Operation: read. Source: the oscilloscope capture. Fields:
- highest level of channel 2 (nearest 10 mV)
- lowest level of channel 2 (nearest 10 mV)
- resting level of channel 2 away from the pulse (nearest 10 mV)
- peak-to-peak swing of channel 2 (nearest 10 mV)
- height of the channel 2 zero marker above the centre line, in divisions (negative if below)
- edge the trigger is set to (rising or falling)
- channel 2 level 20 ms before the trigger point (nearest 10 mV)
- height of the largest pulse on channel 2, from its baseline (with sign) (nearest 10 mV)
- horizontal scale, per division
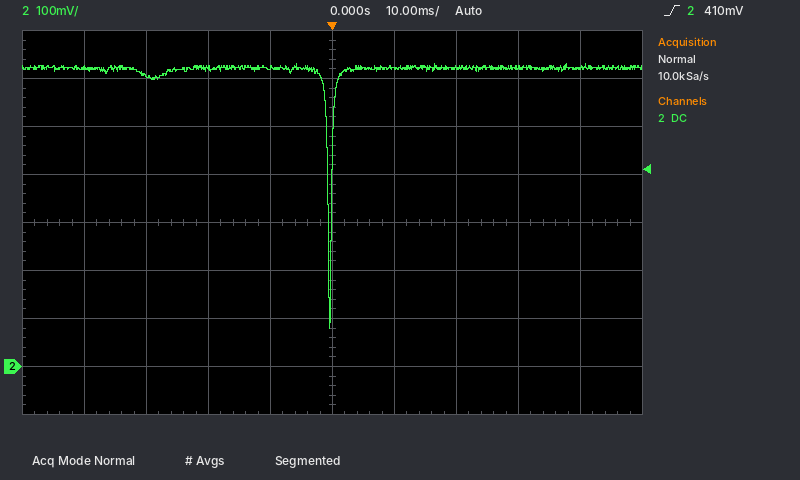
630 mV
80 mV
620 mV
550 mV
-3.0 div
rising
620 mV
-540 mV
10 ms
